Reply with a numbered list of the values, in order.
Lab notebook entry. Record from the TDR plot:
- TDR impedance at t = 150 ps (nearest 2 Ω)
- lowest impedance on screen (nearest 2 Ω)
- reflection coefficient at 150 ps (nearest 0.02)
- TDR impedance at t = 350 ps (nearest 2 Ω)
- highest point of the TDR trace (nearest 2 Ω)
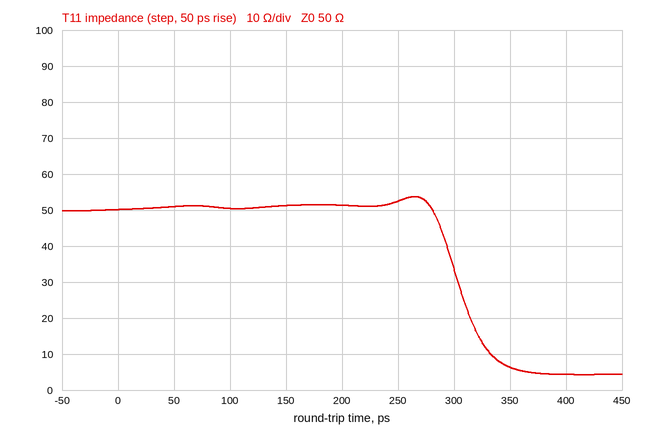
1. 52 Ω
2. 4 Ω
3. +0.02
4. 6 Ω
5. 54 Ω
